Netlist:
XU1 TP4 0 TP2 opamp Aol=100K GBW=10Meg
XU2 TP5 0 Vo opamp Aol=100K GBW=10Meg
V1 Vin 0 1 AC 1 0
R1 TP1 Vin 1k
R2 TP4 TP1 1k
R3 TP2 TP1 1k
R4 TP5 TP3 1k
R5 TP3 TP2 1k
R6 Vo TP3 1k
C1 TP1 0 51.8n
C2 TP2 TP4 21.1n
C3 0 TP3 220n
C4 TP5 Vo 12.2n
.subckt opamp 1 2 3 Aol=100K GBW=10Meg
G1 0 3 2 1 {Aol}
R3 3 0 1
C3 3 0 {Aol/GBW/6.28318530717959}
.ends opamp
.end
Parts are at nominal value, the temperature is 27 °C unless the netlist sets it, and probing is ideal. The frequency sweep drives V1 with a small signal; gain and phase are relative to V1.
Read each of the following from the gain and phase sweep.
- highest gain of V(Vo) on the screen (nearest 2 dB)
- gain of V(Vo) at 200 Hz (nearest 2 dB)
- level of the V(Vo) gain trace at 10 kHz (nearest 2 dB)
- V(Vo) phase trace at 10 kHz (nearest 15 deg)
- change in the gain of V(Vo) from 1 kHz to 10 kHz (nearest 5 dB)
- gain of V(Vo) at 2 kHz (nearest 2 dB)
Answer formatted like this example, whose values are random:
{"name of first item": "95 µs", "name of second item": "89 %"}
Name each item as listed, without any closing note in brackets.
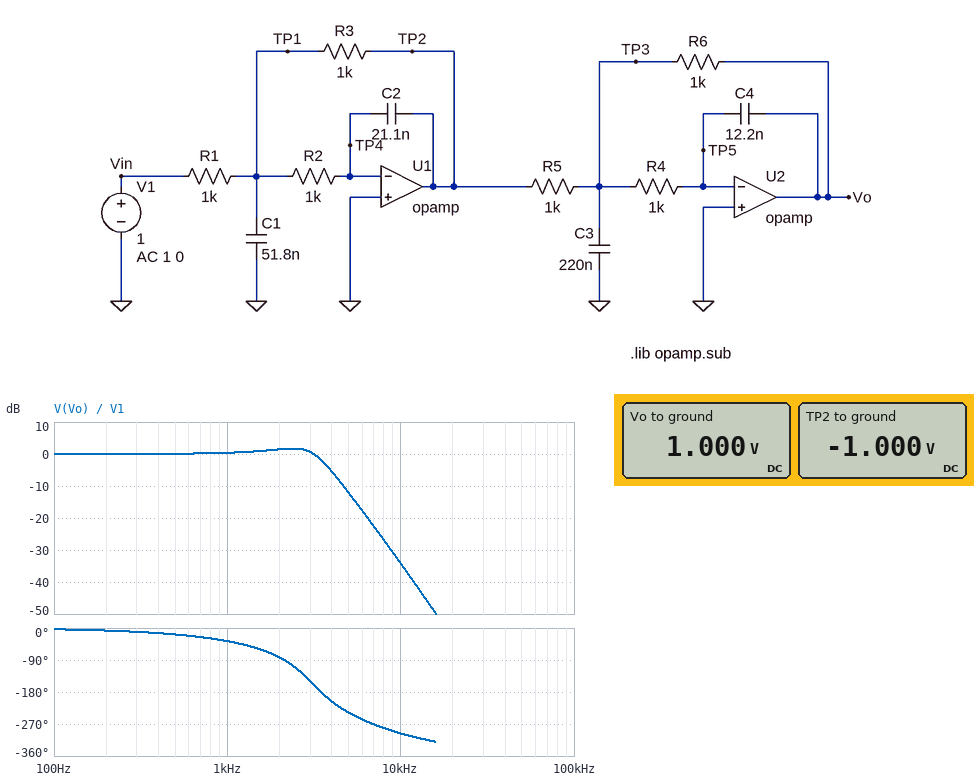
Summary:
{"highest gain of V(Vo) on the screen": "2 dB", "gain of V(Vo) at 200 Hz": "0 dB", "level of the V(Vo) gain trace at 10 kHz": "-34 dB", "V(Vo) phase trace at 10 kHz": "-300 deg", "change in the gain of V(Vo) from 1 kHz to 10 kHz": "-35 dB", "gain of V(Vo) at 2 kHz": "2 dB"}
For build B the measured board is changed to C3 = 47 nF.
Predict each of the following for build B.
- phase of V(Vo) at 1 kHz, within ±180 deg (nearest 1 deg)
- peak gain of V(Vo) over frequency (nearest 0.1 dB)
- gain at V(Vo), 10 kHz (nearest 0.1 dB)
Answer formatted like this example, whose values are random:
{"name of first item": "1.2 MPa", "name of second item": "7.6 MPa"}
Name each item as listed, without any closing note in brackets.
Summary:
{"phase of V(Vo) at 1 kHz, within ±180 deg": "-36 deg", "peak gain of V(Vo) over frequency": "0 dB", "gain at V(Vo), 10 kHz": "-22.7 dB"}
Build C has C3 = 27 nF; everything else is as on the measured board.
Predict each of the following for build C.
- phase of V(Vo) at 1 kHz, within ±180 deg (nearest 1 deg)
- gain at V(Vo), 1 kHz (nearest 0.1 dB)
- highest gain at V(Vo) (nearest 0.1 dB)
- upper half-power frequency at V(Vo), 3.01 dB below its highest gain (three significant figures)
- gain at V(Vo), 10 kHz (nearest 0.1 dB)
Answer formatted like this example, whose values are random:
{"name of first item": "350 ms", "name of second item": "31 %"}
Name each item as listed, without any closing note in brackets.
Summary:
{"phase of V(Vo) at 1 kHz, within ±180 deg": "-36 deg", "gain at V(Vo), 1 kHz": "-0.4 dB", "highest gain at V(Vo)": "0 dB", "upper half-power frequency at V(Vo), 3.01 dB below its highest gain": "2.75 kHz", "gain at V(Vo), 10 kHz": "-21.6 dB"}
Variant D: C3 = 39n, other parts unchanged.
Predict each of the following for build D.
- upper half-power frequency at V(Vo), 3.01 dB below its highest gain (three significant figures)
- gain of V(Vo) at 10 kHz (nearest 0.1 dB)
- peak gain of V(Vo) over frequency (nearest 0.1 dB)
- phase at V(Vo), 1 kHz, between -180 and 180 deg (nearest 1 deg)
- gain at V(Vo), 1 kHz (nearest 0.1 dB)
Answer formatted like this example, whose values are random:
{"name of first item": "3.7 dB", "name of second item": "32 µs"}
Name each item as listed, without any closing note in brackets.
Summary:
{"upper half-power frequency at V(Vo), 3.01 dB below its highest gain": "2.90 kHz", "gain of V(Vo) at 10 kHz": "-22.1 dB", "peak gain of V(Vo) over frequency": "0 dB", "phase at V(Vo), 1 kHz, between -180 and 180 deg": "-36 deg", "gain at V(Vo), 1 kHz": "-0.4 dB"}
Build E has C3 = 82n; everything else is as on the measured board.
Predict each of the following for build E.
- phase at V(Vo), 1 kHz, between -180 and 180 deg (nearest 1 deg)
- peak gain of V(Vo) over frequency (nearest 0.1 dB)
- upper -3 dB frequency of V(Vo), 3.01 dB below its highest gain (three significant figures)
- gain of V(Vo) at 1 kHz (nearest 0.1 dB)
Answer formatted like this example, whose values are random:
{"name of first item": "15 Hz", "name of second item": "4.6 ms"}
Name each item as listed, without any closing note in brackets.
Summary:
{"phase at V(Vo), 1 kHz, between -180 and 180 deg": "-36 deg", "peak gain of V(Vo) over frequency": "0 dB", "upper -3 dB frequency of V(Vo), 3.01 dB below its highest gain": "3.53 kHz", "gain of V(Vo) at 1 kHz": "-0.2 dB"}
